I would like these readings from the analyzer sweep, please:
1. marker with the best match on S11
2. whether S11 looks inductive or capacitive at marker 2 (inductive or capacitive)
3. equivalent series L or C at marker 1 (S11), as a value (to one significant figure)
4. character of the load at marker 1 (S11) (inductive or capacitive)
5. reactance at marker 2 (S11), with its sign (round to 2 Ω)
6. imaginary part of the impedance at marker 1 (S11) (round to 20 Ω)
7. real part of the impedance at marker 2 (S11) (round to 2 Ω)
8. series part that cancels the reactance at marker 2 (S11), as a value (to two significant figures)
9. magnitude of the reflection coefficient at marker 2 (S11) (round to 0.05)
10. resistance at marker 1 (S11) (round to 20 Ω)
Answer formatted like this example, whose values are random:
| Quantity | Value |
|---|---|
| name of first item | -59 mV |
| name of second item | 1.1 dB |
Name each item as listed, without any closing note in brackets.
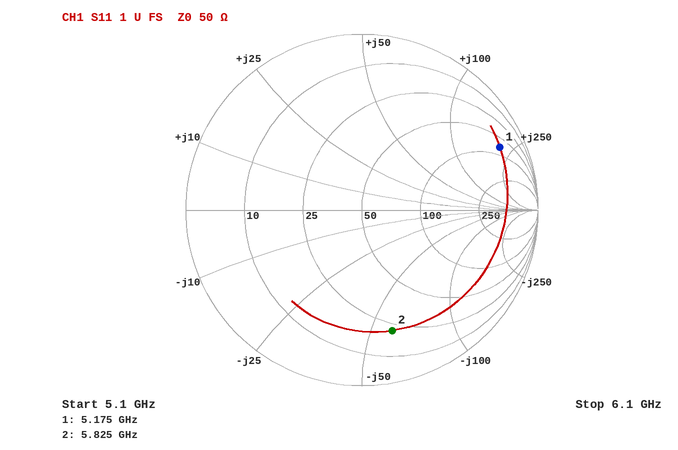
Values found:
| Quantity | Value |
|---|---|
| marker with the best match on S11 | marker 2 |
| whether S11 looks inductive or capacitive at marker 2 | capacitive |
| equivalent series L or C at marker 1 (S11), as a value | 6 nH |
| character of the load at marker 1 (S11) | inductive |
| reactance at marker 2 (S11), with its sign | -60 Ω |
| imaginary part of the impedance at marker 1 (S11) | +200 Ω |
| real part of the impedance at marker 2 (S11) | 22 Ω |
| series part that cancels the reactance at marker 2 (S11), as a value | 1.6 nH |
| magnitude of the reflection coefficient at marker 2 (S11) | 0.70 |
| resistance at marker 1 (S11) | 80 Ω |
